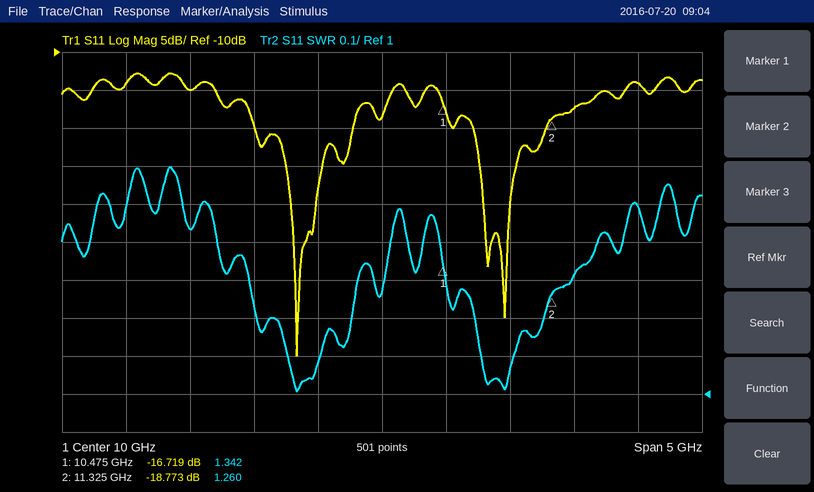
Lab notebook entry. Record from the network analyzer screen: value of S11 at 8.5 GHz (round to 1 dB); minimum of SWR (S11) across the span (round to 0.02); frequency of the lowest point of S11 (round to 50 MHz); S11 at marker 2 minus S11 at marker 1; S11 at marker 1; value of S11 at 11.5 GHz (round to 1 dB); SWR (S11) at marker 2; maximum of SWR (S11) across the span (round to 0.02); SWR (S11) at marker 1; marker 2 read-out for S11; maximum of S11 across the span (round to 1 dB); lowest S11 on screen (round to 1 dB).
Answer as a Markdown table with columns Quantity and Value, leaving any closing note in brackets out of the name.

| Quantity | Value |
|---|---|
| value of S11 at 8.5 GHz | -15 dB |
| minimum of SWR (S11) across the span | 1.00 |
| frequency of the lowest point of S11 | 9.35 GHz |
| S11 at marker 2 minus S11 at marker 1 | -2.054 dB |
| S11 at marker 1 | -16.719 dB |
| value of S11 at 11.5 GHz | -17 dB |
| SWR (S11) at marker 2 | 1.260 |
| maximum of SWR (S11) across the span | 1.60 |
| SWR (S11) at marker 1 | 1.342 |
| marker 2 read-out for S11 | -18.773 dB |
| maximum of S11 across the span | -13 dB |
| lowest S11 on screen | -50 dB |
